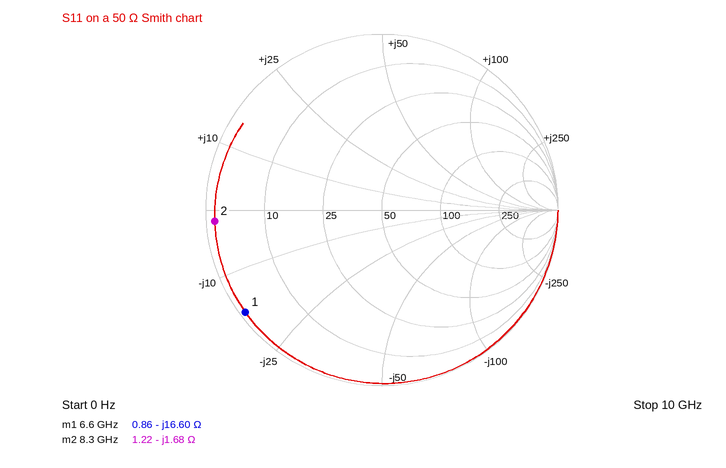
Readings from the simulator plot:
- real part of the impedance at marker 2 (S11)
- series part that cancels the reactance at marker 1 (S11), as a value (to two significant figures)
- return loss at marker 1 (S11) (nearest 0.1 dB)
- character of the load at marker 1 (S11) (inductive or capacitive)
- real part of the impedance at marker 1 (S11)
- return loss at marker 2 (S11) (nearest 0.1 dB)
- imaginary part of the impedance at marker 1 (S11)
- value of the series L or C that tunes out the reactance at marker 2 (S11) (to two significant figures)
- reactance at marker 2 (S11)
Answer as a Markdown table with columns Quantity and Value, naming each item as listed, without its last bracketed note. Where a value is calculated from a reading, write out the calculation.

| Quantity | Value |
|---|---|
| real part of the impedance at marker 2 | 1.22 Ω |
| series part that cancels the reactance at marker 1 (S11), as a value | L = 16.6 Ω/(2π × 6.6 GHz) ≈ 400 pH |
| return loss at marker 1 (S11) | 0.3 dB |
| character of the load at marker 1 (S11) | capacitive |
| real part of the impedance at marker 1 | 0.86 Ω |
| return loss at marker 2 (S11) | 0.4 dB |
| imaginary part of the impedance at marker 1 | -16.60 Ω |
| value of the series L or C that tunes out the reactance at marker 2 (S11) | L = 1.68 Ω/(2π × 8.3 GHz) ≈ 32 pH |
| reactance at marker 2 | -1.68 Ω |
